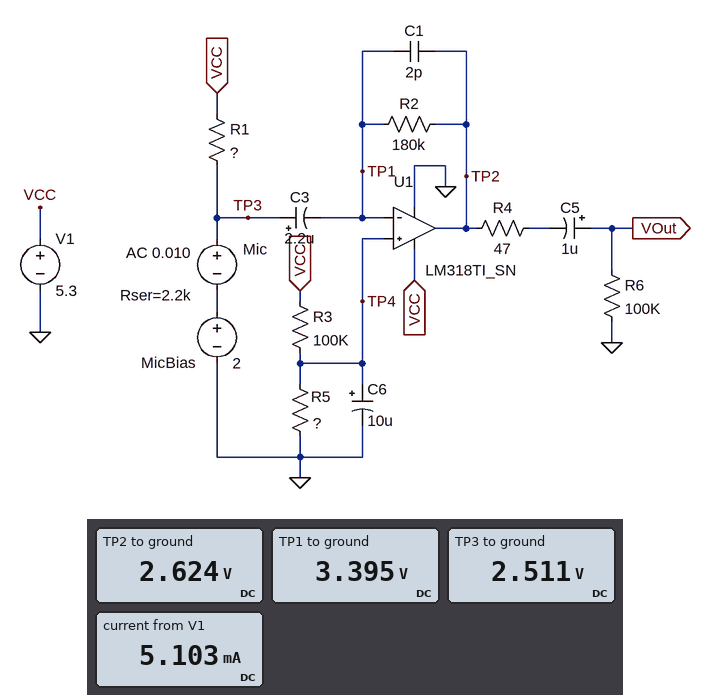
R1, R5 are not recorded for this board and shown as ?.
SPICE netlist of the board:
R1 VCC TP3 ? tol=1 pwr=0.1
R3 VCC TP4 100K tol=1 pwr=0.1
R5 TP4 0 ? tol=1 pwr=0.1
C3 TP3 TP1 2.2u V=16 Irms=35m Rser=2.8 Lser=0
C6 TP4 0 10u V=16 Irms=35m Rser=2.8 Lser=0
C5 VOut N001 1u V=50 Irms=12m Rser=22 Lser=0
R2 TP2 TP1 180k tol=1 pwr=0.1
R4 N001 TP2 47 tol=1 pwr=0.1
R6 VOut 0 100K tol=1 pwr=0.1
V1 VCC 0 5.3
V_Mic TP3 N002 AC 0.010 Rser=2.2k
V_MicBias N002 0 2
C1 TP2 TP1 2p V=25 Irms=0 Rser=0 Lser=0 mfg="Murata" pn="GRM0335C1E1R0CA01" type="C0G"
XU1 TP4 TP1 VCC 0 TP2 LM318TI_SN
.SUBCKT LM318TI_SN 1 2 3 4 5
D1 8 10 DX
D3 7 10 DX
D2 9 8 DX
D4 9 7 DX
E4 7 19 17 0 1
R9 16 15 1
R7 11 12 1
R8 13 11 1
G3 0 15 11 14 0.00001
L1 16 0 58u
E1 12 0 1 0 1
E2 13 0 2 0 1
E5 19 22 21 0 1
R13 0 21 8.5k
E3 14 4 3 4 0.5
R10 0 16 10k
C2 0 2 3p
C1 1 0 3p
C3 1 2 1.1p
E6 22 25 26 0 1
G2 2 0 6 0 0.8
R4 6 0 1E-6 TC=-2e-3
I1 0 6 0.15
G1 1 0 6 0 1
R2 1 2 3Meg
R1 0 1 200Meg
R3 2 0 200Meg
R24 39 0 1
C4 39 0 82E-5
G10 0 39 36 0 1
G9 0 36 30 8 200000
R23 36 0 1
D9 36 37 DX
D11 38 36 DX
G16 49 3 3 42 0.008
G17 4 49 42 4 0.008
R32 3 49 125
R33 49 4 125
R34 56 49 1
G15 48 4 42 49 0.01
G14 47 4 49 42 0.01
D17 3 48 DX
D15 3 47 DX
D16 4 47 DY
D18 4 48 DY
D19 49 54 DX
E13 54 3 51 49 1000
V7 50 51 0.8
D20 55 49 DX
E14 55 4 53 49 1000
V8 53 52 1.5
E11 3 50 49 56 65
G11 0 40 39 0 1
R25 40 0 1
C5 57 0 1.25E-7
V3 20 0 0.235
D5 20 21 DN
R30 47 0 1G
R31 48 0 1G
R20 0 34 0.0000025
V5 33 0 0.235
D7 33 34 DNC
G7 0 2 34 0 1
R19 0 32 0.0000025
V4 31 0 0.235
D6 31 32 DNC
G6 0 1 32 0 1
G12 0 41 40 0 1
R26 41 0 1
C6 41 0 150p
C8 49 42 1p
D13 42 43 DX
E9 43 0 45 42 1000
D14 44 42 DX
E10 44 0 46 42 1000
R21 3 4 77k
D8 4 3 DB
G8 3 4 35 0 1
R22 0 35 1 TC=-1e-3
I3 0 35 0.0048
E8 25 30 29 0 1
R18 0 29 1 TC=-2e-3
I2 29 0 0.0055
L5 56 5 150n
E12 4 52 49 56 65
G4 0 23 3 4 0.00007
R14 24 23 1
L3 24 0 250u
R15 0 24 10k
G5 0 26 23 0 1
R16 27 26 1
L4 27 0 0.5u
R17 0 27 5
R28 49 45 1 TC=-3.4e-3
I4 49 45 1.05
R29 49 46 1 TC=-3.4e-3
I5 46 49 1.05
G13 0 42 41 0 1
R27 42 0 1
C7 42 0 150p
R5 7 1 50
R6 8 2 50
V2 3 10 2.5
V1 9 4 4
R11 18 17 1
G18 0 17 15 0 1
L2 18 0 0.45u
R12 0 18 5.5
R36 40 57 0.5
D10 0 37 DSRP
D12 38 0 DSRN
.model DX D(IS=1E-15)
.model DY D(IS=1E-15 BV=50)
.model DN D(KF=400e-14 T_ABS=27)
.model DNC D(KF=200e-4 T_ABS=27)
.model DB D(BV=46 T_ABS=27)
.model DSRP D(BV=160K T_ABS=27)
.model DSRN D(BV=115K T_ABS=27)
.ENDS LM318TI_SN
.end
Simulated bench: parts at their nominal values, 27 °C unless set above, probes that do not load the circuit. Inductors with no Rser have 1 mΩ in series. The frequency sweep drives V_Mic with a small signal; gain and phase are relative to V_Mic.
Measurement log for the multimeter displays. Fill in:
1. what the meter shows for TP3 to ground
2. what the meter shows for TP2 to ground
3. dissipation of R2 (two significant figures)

2.511 V
2.624 V
3.3 µW
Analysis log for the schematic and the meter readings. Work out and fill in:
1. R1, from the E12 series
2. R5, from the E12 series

12 kΩ
120 kΩ
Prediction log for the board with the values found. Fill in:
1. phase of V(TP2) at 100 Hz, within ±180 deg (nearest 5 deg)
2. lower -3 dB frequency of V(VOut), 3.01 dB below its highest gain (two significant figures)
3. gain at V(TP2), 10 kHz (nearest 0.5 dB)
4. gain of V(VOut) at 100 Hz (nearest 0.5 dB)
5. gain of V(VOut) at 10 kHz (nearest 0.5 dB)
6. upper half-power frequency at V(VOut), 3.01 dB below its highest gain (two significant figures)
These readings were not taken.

-160 deg
39 Hz
38.0 dB
37.5 dB
38.0 dB
120 kHz
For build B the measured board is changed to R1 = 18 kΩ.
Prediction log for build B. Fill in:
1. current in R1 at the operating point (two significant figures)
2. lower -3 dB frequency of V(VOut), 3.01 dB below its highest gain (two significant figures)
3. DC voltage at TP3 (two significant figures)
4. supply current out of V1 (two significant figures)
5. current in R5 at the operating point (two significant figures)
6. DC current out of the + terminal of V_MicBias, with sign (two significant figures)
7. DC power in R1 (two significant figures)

160 µA
37 Hz
2.4 V
5.0 mA
28 µA
-160 µA
480 µW
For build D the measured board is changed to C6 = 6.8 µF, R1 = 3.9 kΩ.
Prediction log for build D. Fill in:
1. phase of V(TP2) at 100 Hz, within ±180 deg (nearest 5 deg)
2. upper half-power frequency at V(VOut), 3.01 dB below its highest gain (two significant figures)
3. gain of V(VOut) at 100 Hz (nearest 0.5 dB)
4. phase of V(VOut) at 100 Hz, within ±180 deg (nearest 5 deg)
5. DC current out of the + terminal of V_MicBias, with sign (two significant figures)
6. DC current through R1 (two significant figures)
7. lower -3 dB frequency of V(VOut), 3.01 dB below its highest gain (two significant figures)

-155 deg
110 kHz
37.0 dB
-150 deg
-540 µA
540 µA
51 Hz
